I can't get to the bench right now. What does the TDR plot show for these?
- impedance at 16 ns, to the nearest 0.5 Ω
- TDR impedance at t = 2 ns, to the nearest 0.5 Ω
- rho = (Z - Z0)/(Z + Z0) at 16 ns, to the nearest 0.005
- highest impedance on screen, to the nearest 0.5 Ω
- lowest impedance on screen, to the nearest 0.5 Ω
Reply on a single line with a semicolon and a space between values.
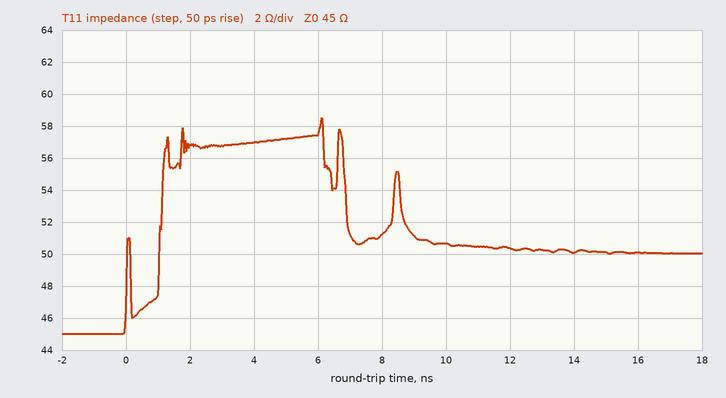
50.0 Ω; 57.0 Ω; +0.055; 58.5 Ω; 45.0 Ω
